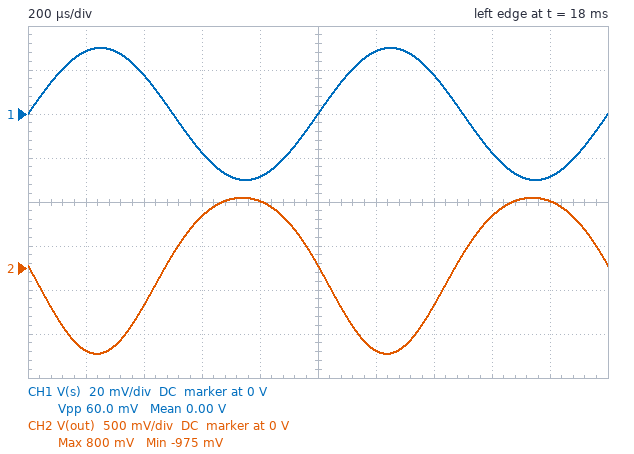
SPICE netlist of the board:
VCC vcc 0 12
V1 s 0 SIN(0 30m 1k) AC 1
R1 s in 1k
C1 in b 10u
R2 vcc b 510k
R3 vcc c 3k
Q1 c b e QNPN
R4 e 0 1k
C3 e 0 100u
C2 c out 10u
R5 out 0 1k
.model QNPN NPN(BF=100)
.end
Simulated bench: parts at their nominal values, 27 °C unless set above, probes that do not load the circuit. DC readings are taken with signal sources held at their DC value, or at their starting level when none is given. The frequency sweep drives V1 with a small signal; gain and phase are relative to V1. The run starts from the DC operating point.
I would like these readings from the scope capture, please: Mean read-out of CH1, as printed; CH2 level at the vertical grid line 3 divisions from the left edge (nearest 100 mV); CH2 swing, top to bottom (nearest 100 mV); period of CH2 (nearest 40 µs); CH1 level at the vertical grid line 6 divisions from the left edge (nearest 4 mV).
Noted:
0.00 V
600 mV
1.8 V
1.00 ms
28 mV
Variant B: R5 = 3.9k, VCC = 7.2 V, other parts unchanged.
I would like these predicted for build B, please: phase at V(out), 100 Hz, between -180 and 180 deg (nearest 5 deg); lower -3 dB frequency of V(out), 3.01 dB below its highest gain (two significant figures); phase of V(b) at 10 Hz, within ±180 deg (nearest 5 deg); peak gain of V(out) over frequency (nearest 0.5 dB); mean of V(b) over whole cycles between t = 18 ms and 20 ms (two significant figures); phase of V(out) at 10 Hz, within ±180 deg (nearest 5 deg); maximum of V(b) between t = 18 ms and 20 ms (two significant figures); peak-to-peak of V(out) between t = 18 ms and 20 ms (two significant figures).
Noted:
-150 deg
53 Hz
0 deg
34.0 dB
1.8 V
-95 deg
1.9 V
2.7 V
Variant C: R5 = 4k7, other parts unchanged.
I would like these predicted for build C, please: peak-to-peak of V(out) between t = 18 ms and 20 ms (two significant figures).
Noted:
4.3 V
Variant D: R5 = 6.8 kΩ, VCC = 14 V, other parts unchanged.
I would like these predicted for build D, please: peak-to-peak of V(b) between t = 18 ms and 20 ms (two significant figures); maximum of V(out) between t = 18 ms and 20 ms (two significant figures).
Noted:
34 mV
2.5 V
